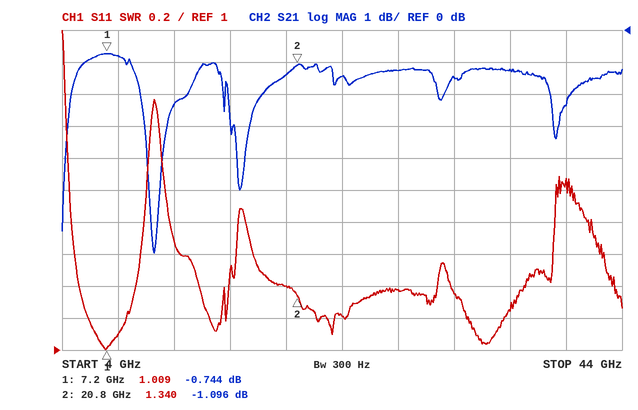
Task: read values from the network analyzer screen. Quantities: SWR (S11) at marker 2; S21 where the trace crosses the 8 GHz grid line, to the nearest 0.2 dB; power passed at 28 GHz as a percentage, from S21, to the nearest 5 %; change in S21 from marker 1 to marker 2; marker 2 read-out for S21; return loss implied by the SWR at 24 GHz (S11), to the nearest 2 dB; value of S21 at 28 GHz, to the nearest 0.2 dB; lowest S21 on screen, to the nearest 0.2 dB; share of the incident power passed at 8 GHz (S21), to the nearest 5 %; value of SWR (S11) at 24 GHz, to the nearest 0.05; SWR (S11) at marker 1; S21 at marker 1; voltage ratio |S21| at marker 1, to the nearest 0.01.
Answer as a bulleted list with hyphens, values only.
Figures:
- 1.340
- -0.8 dB
- 75 %
- -0.352 dB
- -1.096 dB
- 20 dB
- -1.2 dB
- -7.0 dB
- 85 %
- 1.20
- 1.009
- -0.744 dB
- 0.92
